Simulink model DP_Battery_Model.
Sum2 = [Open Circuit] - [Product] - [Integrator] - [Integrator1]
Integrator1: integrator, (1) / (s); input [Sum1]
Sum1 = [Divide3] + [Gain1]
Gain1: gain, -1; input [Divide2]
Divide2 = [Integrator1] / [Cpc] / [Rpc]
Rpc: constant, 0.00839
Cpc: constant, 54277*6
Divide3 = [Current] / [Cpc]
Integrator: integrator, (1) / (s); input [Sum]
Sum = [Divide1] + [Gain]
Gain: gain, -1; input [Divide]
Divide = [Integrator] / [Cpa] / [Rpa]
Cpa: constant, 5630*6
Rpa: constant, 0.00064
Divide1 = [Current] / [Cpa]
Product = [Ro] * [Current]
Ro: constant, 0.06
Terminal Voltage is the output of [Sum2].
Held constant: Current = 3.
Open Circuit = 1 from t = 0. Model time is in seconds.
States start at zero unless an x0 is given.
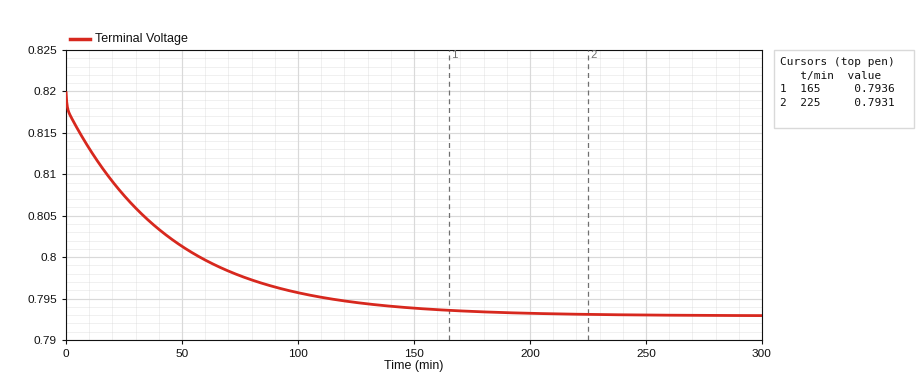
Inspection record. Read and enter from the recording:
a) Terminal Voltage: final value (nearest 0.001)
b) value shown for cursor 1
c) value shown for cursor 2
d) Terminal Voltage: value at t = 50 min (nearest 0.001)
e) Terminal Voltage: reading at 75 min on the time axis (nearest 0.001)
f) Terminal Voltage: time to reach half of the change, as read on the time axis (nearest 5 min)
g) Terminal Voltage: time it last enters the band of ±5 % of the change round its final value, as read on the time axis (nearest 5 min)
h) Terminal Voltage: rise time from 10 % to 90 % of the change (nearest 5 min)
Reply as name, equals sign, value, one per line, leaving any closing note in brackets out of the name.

Terminal Voltage: final value = 0.793
value shown for cursor 1 = 0.7936
value shown for cursor 2 = 0.7931
Terminal Voltage: value at t = 50 min = 0.801
Terminal Voltage: reading at 75 min on the time axis = 0.798
Terminal Voltage: time to reach half of the change, as read on the time axis = 30 min
Terminal Voltage: time it last enters the band of ±5 % of the change round its final value, as read on the time axis = 135 min
Terminal Voltage: rise time from 10 % to 90 % of the change = 100 min
